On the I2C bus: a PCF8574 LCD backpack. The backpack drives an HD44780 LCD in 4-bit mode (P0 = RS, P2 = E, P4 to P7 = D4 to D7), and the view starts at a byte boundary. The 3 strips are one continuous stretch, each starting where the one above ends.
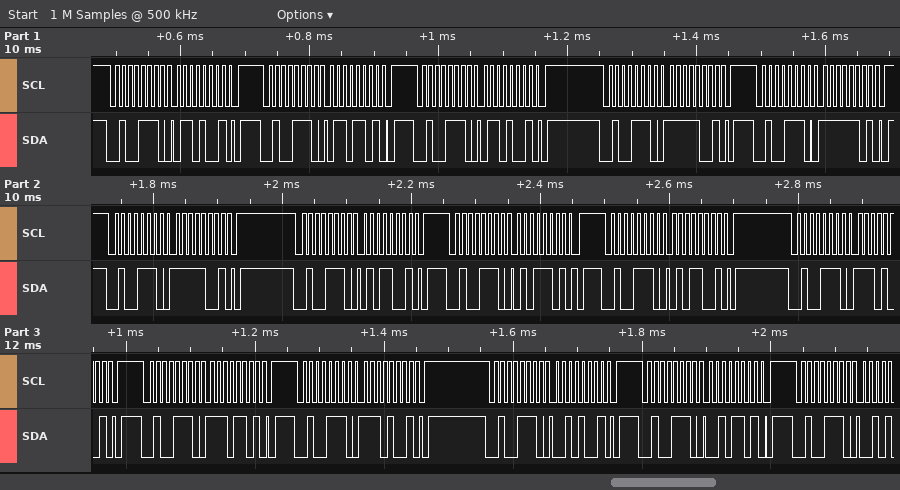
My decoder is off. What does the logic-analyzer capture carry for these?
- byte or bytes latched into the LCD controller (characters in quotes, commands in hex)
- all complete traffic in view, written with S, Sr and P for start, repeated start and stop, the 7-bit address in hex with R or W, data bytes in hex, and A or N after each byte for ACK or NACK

'o' '^'
S 27W A 69 A P S 27W A 6D A P S 27W A 69 A P S 27W A F9 A P S 27W A FD A P S 27W A F9 A P S 27W A 59 A P S 27W A 5D A P S 27W A 59 A P S 27W A E9 A P S 27W A ED A P S 27W A E9 A P S 27W A 29 A P S 27W A 2D A P S 27W A
